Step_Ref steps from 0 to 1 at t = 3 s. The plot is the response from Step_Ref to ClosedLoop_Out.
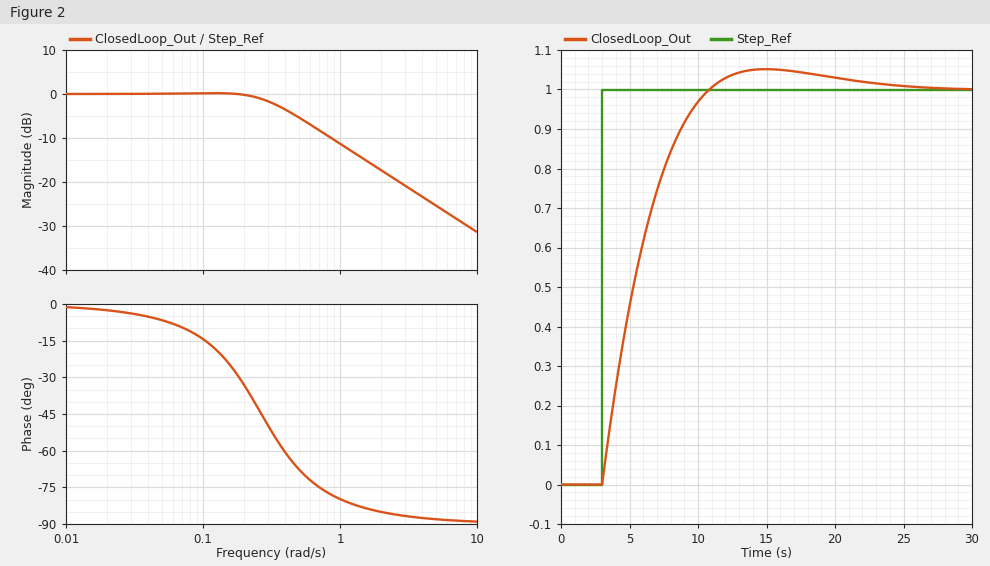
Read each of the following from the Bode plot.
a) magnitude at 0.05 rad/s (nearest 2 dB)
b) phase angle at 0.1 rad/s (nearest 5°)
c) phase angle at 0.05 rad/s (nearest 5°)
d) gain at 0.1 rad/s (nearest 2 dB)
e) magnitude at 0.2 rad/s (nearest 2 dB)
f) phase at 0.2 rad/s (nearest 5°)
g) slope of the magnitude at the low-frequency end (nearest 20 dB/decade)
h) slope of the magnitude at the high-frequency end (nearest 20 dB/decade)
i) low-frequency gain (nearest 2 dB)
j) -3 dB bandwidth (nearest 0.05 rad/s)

0 dB
-15°
-5°
0 dB
0 dB
-35°
0 dB/decade
-20 dB/decade
0 dB
0.35 rad/s
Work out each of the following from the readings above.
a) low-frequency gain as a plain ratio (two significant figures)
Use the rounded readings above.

1.0
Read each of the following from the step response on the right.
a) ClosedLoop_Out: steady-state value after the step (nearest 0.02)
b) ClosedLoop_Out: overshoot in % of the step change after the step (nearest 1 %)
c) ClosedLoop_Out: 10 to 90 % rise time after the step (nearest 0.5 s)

1.00
5 %
5.5 s
